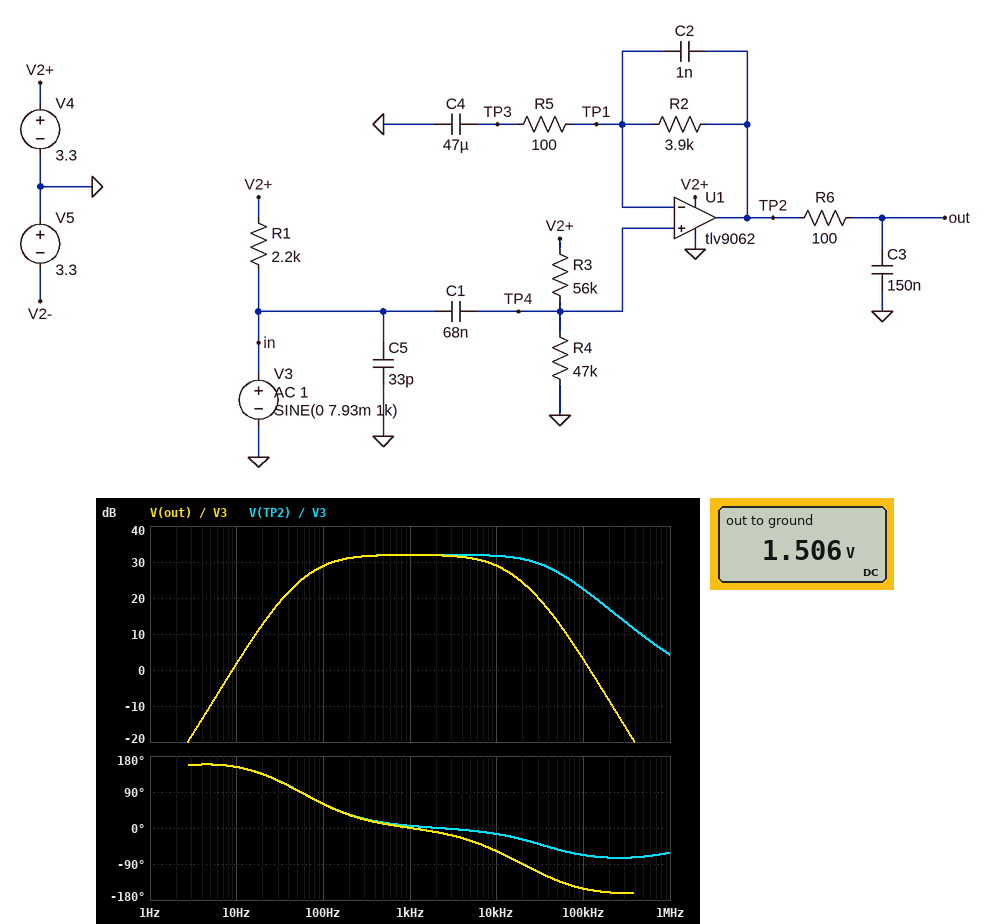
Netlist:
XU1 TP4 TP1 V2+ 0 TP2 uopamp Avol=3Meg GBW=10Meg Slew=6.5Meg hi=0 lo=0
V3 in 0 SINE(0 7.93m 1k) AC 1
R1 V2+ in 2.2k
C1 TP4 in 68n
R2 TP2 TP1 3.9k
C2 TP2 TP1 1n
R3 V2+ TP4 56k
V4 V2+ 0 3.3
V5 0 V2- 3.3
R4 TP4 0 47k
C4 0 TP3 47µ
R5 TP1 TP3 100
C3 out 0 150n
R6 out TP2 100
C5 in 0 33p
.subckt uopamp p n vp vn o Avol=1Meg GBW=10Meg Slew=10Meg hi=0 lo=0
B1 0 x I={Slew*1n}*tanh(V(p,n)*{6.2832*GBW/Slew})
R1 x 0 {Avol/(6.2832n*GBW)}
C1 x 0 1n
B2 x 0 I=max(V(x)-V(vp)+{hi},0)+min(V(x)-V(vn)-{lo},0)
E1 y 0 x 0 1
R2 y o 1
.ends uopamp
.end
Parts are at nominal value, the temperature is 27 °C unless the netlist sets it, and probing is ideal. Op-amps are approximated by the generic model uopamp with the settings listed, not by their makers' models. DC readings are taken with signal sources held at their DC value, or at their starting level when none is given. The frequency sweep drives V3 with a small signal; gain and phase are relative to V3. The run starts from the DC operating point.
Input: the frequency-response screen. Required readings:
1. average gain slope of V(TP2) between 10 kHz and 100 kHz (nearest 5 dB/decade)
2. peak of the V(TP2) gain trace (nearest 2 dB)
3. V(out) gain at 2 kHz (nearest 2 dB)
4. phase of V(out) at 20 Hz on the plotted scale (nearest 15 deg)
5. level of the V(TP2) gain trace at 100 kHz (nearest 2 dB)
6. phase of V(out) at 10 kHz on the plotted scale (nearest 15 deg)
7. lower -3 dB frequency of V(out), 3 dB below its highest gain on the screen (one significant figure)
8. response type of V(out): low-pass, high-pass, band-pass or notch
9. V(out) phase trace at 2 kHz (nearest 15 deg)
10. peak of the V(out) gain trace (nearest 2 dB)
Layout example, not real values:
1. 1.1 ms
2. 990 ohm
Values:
1. -10 dB/decade
2. 32 dB
3. 32 dB
4. 135 deg
5. 22 dB
6. -60 deg
7. 100 Hz
8. band-pass
9. -15 deg
10. 32 dB
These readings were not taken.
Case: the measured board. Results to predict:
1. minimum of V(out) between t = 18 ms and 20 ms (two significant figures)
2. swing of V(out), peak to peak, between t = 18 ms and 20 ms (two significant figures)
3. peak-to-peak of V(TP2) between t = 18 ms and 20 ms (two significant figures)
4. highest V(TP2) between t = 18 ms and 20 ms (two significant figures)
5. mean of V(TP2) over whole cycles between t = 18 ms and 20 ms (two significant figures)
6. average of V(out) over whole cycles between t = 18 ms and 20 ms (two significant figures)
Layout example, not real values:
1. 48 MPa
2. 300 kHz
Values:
1. 1.2 V
2. 630 mV
3. 630 mV
4. 1.8 V
5. 1.5 V
6. 1.5 V
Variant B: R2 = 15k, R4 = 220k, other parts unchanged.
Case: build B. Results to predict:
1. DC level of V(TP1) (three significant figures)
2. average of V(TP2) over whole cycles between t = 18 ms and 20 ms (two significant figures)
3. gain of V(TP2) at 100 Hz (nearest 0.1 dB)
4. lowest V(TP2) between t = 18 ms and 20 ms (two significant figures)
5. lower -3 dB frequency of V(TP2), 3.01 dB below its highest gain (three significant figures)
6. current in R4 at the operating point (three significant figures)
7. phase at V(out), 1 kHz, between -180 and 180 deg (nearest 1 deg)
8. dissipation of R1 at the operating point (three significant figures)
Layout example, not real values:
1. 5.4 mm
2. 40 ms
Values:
1. 2.63 V
2. 2.6 V
3. 42.1 dB
4. 1.6 V
5. 66.9 Hz
6. 12.0 µA
7. -7 deg
8. 4.95 mW
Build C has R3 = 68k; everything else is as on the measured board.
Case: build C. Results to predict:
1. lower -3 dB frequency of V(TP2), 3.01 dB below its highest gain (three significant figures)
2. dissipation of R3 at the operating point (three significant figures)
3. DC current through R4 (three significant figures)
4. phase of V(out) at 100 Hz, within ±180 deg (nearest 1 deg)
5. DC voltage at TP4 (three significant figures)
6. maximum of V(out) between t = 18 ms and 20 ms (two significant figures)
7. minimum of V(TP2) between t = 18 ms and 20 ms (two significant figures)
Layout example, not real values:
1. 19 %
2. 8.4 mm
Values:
1. 95.1 Hz
2. 56.0 µW
3. 28.7 µA
4. 58 deg
5. 1.35 V
6. 1.7 V
7. 1.0 V
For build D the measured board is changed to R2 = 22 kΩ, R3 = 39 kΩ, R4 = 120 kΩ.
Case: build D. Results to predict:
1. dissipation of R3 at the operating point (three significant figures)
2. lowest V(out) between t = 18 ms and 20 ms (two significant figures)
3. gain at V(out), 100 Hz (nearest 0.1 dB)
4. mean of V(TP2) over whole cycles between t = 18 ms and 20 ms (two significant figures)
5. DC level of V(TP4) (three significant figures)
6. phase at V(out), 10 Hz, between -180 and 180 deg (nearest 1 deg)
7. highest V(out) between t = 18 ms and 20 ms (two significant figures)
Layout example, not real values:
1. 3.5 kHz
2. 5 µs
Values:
1. 16.8 µW
2. 1.1 V
3. 44.3 dB
4. 2.5 V
5. 2.49 V
6. 155 deg
7. 3.3 V
